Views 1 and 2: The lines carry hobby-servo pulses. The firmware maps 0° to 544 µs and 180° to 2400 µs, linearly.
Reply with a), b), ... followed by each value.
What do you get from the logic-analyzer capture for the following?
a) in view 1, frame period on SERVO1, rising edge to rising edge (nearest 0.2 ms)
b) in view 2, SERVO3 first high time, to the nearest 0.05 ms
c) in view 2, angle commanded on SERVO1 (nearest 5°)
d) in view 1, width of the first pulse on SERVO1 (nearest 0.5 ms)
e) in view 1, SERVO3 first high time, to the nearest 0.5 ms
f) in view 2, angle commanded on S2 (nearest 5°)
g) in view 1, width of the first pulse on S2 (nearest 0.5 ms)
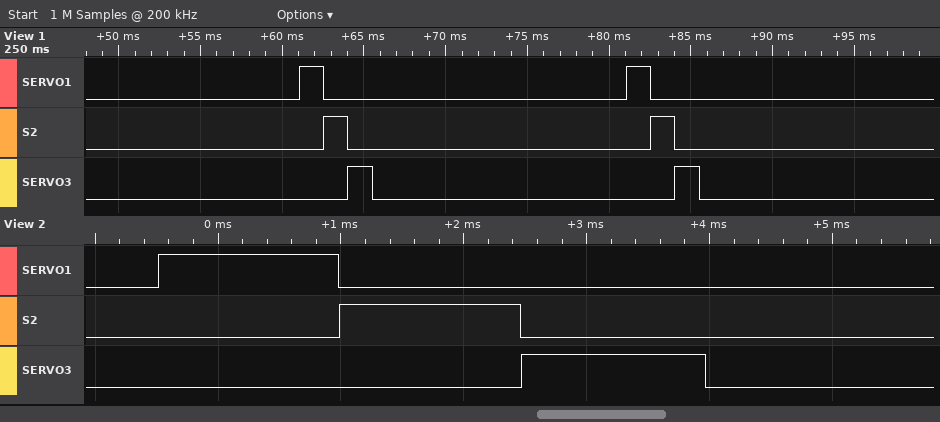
a) 20.0 ms
b) 1.50 ms
c) 90°
d) 1.5 ms
e) 1.5 ms
f) 90°
g) 1.5 ms
